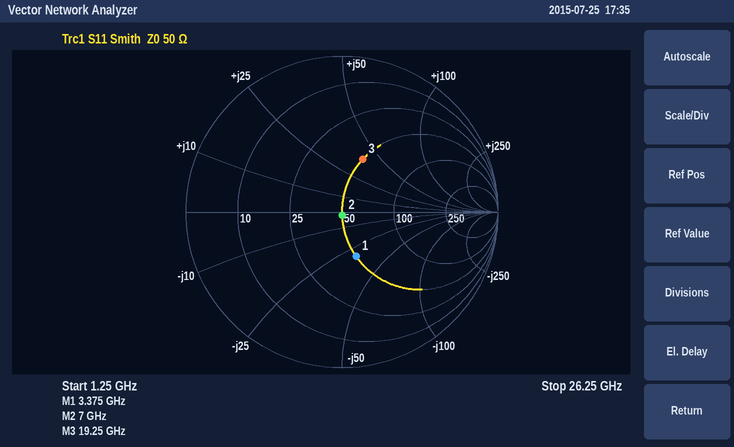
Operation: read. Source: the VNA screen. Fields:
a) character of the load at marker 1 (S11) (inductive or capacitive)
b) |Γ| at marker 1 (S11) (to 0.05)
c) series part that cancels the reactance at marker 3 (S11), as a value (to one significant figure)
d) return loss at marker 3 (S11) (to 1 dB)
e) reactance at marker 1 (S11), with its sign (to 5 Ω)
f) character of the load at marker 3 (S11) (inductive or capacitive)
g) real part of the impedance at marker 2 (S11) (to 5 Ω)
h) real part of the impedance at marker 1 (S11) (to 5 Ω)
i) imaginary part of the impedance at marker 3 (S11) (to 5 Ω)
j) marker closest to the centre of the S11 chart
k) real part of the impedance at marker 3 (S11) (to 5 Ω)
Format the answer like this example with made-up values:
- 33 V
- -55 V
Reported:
- capacitive
- 0.30
- 200 fF
- 9 dB
- -30 Ω
- inductive
- 50 Ω
- 50 Ω
- +40 Ω
- marker 2
- 50 Ω
